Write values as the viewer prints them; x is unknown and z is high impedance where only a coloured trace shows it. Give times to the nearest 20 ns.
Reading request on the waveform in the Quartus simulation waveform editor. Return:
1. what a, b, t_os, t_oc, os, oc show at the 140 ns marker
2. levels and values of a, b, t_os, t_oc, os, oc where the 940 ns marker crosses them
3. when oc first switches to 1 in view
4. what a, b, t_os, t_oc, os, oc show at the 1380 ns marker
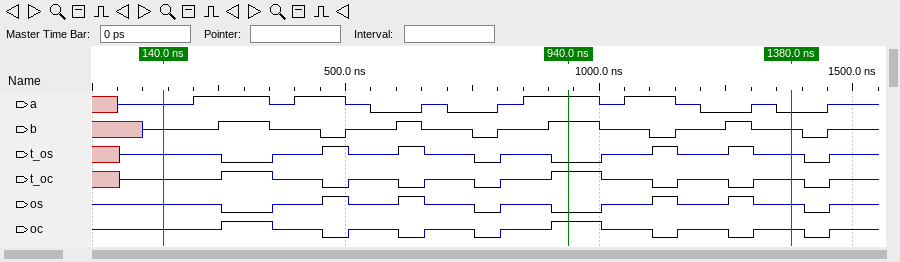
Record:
a=z, b=z, t_os=z, t_oc=z, os=z, oc=z
a=1, b=1, t_os=0, t_oc=1, os=0, oc=1
260 ns
a=0, b=z, t_os=z, t_oc=z, os=z, oc=z
